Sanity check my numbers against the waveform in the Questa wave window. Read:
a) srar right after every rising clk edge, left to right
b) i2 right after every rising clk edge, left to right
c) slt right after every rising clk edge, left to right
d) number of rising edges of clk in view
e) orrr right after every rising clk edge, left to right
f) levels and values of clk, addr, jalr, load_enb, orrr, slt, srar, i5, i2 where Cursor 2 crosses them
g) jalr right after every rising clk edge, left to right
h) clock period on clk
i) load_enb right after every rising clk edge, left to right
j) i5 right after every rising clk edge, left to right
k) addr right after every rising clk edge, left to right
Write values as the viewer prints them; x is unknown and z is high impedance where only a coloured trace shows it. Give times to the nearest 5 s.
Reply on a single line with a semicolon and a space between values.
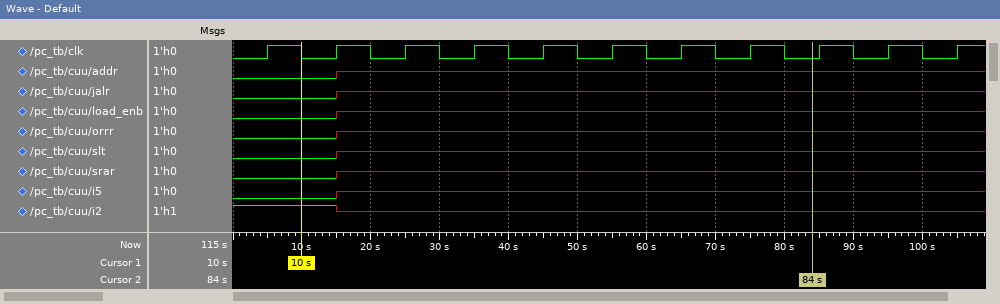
0 x x x x x x x x x x; 1 x x x x x x x x x x; 0 x x x x x x x x x x; 11; 0 x x x x x x x x x x; clk=0, addr=x, jalr=x, load_enb=x, orrr=x, slt=x, srar=x, i5=x, i2=x; 0 x x x x x x x x x x; 10 s; 0 x x x x x x x x x x; 0 x x x x x x x x x x; 0 x x x x x x x x x x
